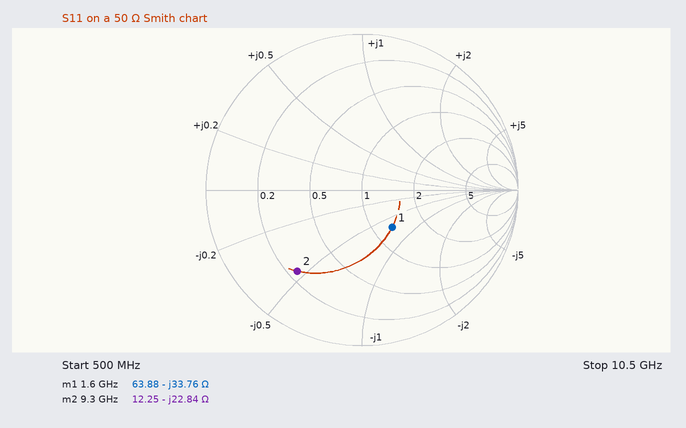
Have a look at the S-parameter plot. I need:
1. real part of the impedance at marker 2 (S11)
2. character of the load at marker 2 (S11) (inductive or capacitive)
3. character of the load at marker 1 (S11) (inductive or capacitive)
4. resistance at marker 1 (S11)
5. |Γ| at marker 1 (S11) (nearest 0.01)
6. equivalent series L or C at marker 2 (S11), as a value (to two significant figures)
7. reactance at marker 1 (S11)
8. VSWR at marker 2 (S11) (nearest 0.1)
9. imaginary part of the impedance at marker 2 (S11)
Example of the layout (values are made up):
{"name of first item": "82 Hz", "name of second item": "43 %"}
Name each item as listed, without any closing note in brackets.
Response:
{"real part of the impedance at marker 2": "12.25 Ω", "character of the load at marker 2 (S11)": "capacitive", "character of the load at marker 1 (S11)": "capacitive", "resistance at marker 1": "63.88 Ω", "|Γ| at marker 1 (S11)": "0.31", "equivalent series L or C at marker 2 (S11), as a value": "750 fF", "reactance at marker 1": "-33.76 Ω", "VSWR at marker 2 (S11)": "5.0", "imaginary part of the impedance at marker 2": "-22.84 Ω"}
